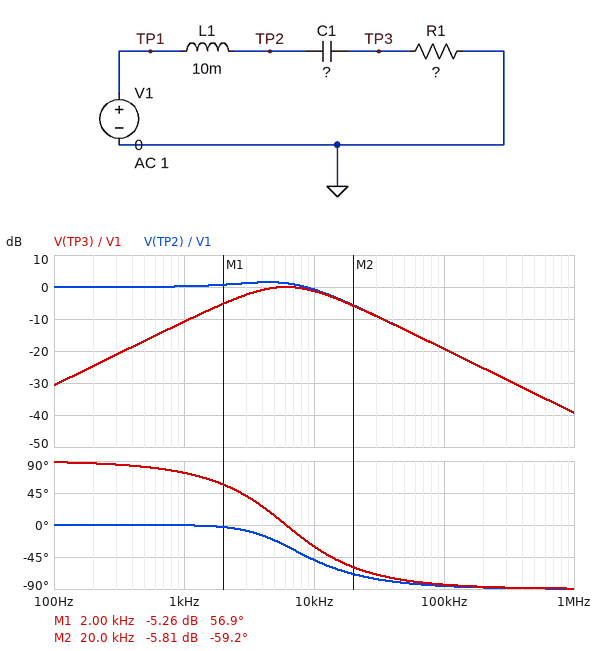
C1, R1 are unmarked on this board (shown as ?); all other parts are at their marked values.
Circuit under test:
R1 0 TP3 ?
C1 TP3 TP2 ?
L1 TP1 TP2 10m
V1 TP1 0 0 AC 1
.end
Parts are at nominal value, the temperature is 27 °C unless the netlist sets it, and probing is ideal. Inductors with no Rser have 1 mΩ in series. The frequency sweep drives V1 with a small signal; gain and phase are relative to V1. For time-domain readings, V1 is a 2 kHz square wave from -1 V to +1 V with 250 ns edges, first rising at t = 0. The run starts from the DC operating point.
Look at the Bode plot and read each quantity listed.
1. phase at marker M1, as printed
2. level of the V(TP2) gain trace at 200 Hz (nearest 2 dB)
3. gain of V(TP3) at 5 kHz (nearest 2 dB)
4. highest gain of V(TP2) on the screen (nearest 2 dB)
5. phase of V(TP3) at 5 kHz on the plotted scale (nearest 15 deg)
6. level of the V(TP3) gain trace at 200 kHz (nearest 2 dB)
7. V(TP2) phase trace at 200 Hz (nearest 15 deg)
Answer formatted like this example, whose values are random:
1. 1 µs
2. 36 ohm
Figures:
1. 56.9 deg
2. 0 dB
3. 0 dB
4. 2 dB
5. 15 deg
6. -26 dB
7. 0 deg
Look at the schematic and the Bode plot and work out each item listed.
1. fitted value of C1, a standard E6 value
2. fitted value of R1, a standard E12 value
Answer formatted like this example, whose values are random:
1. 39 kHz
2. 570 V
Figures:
1. 68 nF
2. 680 Ω
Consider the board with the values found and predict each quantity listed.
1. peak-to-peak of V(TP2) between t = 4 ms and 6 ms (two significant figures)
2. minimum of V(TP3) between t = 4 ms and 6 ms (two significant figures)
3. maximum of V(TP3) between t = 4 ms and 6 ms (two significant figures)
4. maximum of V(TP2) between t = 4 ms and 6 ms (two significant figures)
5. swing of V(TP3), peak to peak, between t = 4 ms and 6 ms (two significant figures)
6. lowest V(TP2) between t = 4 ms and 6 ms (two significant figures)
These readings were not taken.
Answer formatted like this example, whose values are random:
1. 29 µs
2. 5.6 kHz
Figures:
1. 2.6 V
2. -1.4 V
3. 1.4 V
4. 1.3 V
5. 2.8 V
6. -1.3 V
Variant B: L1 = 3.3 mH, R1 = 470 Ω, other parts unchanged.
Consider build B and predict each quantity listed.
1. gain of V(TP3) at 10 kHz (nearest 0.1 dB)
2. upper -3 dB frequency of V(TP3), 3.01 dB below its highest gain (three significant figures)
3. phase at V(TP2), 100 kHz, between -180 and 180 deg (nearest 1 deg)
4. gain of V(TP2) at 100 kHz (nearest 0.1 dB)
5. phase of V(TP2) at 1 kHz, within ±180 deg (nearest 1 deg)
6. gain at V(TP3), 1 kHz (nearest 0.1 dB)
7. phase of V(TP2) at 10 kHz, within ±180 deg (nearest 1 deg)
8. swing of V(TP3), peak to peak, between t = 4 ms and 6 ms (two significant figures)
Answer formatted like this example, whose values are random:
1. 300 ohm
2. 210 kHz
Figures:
1. 0 dB
2. 26.9 kHz
3. -80 deg
4. -13.0 dB
5. 0 deg
6. -14.0 dB
7. -23 deg
8. 3.0 V
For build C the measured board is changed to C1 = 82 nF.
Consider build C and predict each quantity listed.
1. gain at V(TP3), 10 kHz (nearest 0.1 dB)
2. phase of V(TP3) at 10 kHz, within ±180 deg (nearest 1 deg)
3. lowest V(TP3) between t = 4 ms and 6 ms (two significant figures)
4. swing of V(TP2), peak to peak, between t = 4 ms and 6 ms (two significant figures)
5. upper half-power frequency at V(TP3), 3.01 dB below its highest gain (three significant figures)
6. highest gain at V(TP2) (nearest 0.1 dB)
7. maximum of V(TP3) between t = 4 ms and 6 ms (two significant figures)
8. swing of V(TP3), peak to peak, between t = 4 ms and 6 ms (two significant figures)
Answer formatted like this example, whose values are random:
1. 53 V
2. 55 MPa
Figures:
1. -1.5 dB
2. -33 deg
3. -1.5 V
4. 2.6 V
5. 13.2 kHz
6. 1.3 dB
7. 1.5 V
8. 2.9 V
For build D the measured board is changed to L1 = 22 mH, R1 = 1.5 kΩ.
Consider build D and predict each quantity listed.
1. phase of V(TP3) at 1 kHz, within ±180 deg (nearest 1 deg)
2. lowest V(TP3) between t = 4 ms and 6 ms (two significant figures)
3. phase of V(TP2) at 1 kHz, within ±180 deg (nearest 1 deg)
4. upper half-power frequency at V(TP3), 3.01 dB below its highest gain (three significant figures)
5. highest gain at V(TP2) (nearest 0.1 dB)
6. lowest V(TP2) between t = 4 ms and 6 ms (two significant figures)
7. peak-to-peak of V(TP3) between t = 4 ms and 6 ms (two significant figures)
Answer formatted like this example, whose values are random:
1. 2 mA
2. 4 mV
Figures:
1. 56 deg
2. -1.5 V
3. -2 deg
4. 12.2 kHz
5. 0.8 dB
6. -1.2 V
7. 3.0 V
